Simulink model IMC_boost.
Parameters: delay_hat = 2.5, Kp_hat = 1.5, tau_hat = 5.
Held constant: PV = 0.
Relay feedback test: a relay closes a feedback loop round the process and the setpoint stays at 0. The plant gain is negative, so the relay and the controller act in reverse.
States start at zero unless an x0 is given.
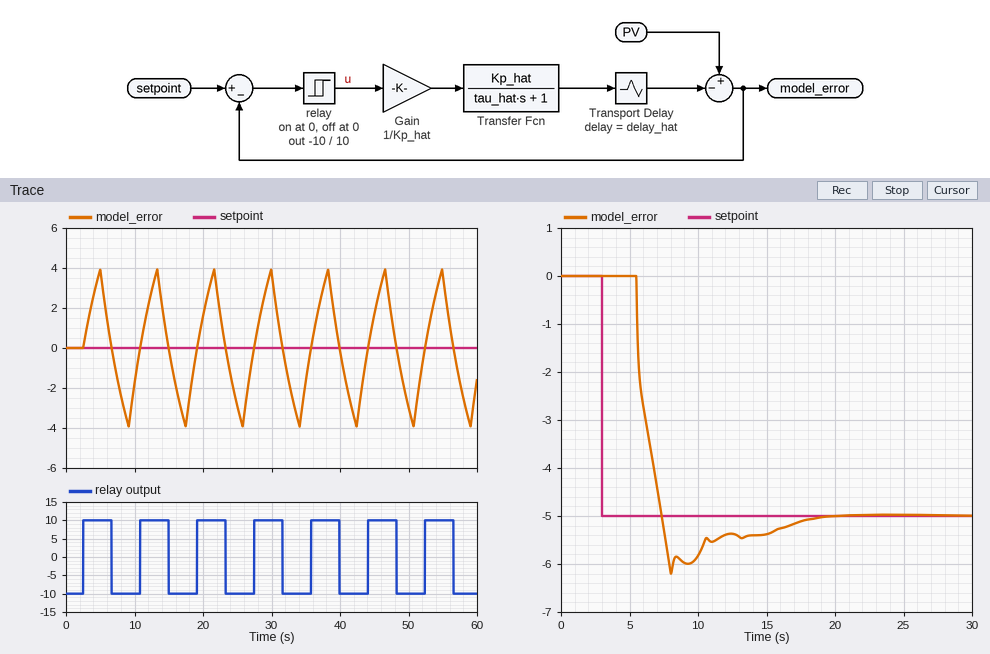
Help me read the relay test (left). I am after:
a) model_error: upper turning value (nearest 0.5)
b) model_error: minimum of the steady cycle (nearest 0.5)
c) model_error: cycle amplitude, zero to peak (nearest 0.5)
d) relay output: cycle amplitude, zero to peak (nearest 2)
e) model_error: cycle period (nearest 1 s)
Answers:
4.0
-4.0
4.0
10
8 s
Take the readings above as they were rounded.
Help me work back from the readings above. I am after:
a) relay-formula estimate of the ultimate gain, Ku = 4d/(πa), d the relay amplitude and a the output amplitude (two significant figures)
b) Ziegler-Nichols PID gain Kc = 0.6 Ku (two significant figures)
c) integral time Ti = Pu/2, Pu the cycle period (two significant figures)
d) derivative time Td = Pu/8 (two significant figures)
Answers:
3.2
1.9
4.0 s
1.0 s
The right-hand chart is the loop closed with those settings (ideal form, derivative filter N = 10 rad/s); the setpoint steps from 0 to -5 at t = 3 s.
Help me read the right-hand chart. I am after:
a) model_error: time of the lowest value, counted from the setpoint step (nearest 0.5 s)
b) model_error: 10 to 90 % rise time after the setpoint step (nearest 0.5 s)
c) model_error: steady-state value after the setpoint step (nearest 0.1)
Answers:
5.0 s
1.5 s
-5.0
